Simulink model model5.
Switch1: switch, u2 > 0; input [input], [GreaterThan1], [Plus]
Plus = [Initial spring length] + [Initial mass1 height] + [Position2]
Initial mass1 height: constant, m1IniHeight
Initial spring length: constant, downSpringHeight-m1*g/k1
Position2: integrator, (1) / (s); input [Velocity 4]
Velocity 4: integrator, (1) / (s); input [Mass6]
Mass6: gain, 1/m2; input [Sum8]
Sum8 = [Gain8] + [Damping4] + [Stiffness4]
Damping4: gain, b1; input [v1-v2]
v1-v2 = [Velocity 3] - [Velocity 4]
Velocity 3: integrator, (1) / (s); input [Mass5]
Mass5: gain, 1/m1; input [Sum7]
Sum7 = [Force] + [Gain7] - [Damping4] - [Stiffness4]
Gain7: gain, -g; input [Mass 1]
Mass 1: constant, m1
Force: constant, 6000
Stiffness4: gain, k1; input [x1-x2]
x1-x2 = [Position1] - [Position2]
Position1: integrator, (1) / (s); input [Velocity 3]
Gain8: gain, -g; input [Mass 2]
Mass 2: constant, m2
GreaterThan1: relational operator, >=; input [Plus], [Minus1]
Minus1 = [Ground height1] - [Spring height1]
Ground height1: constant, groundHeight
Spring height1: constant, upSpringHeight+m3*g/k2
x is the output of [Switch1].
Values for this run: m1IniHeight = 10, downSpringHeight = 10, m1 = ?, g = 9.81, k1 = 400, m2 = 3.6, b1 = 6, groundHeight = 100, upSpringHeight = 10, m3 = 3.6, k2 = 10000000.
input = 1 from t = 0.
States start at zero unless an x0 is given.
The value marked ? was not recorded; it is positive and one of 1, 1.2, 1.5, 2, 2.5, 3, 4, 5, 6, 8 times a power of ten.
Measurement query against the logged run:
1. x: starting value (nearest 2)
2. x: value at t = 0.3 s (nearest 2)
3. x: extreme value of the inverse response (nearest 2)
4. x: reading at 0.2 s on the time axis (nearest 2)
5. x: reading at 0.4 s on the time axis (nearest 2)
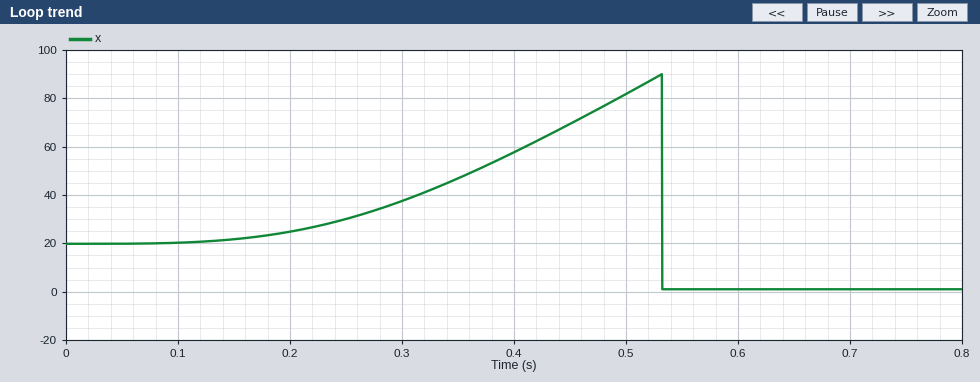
20
38
90
24
58
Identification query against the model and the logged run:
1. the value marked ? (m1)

8
